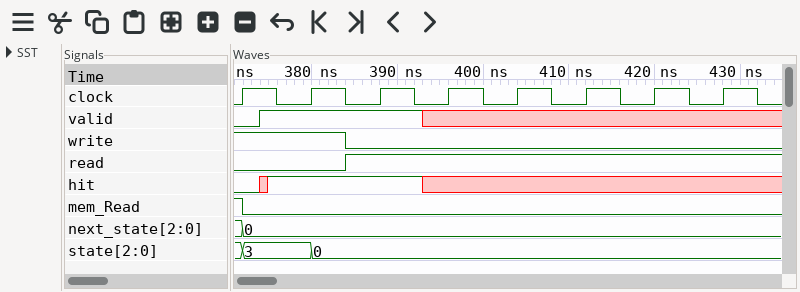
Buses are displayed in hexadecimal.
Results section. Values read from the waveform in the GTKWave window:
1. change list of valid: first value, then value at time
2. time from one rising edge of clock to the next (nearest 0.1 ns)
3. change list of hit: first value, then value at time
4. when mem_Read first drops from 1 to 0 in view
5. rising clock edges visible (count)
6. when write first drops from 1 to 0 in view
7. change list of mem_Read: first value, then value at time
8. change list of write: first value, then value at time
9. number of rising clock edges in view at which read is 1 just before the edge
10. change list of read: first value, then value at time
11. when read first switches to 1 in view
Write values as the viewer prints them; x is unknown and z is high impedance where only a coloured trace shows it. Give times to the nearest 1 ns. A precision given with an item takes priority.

0, 1 at 374 ns, x at 393 ns
8 ns
0, x at 374 ns, 1 at 375 ns, x at 393 ns
372 ns
8
384 ns
1, 0 at 372 ns
1, 0 at 384 ns
6
0, 1 at 384 ns
384 ns
